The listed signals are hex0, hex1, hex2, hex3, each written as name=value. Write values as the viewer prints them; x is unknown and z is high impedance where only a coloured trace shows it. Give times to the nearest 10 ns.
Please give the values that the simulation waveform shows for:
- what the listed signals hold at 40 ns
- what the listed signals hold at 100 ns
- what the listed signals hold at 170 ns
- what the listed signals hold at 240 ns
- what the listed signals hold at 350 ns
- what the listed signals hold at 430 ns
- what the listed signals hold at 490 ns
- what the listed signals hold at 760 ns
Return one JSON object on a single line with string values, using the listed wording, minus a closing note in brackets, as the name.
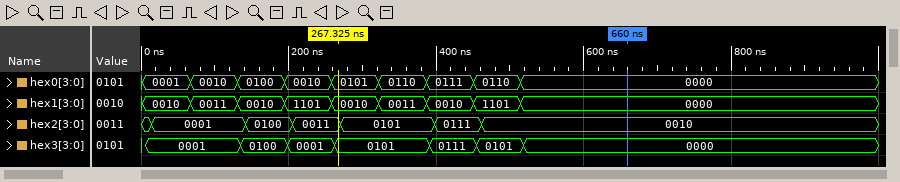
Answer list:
{"what the listed signals hold at 40 ns": "hex0=0001, hex1=0010, hex2=0001, hex3=0001", "what the listed signals hold at 100 ns": "hex0=0010, hex1=0011, hex2=0001, hex3=0001", "what the listed signals hold at 170 ns": "hex0=0100, hex1=0010, hex2=0100, hex3=0100", "what the listed signals hold at 240 ns": "hex0=0010, hex1=1101, hex2=0011, hex3=0001", "what the listed signals hold at 350 ns": "hex0=0110, hex1=0011, hex2=0101, hex3=0101", "what the listed signals hold at 430 ns": "hex0=0111, hex1=0010, hex2=0111, hex3=0111", "what the listed signals hold at 490 ns": "hex0=0110, hex1=1101, hex2=0010, hex3=0101", "what the listed signals hold at 760 ns": "hex0=0000, hex1=0000, hex2=0010, hex3=0000"}
